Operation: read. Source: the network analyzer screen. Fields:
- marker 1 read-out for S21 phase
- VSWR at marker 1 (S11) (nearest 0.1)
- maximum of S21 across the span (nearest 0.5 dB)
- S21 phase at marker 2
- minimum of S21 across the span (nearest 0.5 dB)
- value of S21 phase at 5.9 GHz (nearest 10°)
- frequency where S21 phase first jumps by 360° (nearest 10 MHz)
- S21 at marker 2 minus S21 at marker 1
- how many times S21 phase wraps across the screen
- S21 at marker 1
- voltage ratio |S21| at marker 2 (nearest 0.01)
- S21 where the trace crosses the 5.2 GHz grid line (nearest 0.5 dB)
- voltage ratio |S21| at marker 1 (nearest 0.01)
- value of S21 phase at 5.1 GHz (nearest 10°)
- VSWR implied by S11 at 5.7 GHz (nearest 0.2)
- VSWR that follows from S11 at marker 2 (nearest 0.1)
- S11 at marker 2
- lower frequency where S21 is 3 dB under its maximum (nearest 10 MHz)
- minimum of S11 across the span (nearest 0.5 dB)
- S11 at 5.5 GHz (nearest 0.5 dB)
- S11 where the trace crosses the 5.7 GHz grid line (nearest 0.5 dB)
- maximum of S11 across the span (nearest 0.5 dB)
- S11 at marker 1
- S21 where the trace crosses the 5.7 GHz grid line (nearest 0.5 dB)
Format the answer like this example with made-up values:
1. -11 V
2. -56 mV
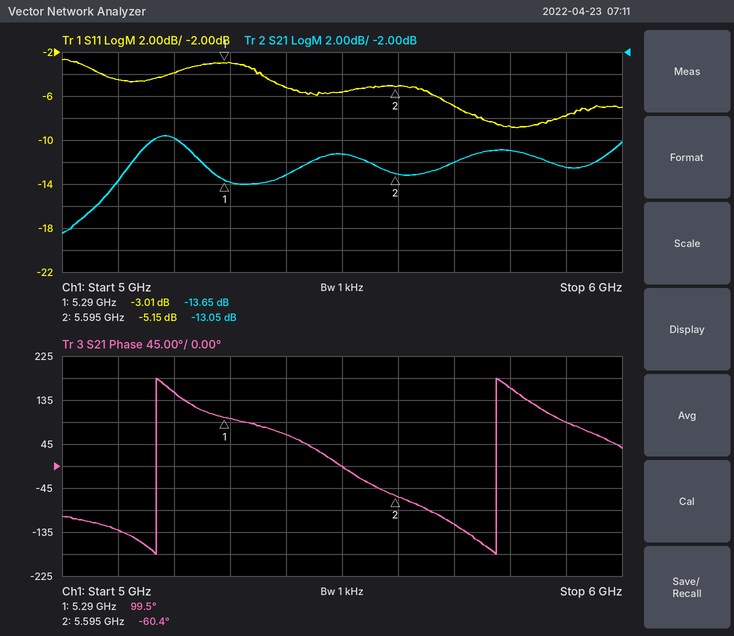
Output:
1. 99.5°
2. 5.8
3. -9.5 dB
4. -60.4°
5. -18.5 dB
6. 90°
7. 5.17 GHz
8. 0.60 dB
9. 2
10. -13.65 dB
11. 0.22
12. -10.0 dB
13. 0.21
14. -130°
15. 2.6
16. 3.5
17. -5.15 dB
18. 5.12 GHz
19. -9.0 dB
20. -5.5 dB
21. -7.0 dB
22. -2.5 dB
23. -3.01 dB
24. -12.0 dB
